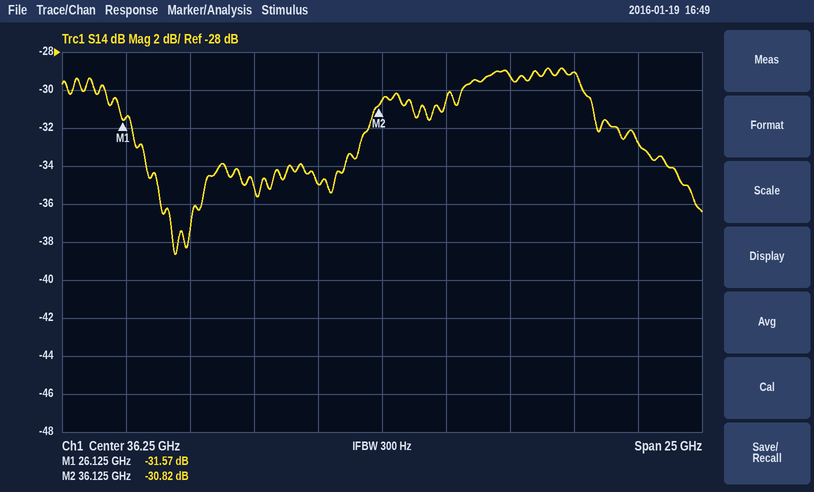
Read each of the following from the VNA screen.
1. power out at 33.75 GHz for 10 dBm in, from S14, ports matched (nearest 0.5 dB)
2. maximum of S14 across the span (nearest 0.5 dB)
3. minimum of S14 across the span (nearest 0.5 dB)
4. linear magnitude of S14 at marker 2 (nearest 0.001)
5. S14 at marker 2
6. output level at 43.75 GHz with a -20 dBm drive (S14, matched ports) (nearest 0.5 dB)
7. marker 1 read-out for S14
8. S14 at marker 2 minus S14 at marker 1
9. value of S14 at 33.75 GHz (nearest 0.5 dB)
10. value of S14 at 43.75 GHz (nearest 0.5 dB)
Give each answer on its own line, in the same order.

-25.0 dBm
-29.0 dB
-38.5 dB
0.029
-30.82 dB
-49.0 dBm
-31.57 dB
0.75 dB
-35.0 dB
-29.0 dB
